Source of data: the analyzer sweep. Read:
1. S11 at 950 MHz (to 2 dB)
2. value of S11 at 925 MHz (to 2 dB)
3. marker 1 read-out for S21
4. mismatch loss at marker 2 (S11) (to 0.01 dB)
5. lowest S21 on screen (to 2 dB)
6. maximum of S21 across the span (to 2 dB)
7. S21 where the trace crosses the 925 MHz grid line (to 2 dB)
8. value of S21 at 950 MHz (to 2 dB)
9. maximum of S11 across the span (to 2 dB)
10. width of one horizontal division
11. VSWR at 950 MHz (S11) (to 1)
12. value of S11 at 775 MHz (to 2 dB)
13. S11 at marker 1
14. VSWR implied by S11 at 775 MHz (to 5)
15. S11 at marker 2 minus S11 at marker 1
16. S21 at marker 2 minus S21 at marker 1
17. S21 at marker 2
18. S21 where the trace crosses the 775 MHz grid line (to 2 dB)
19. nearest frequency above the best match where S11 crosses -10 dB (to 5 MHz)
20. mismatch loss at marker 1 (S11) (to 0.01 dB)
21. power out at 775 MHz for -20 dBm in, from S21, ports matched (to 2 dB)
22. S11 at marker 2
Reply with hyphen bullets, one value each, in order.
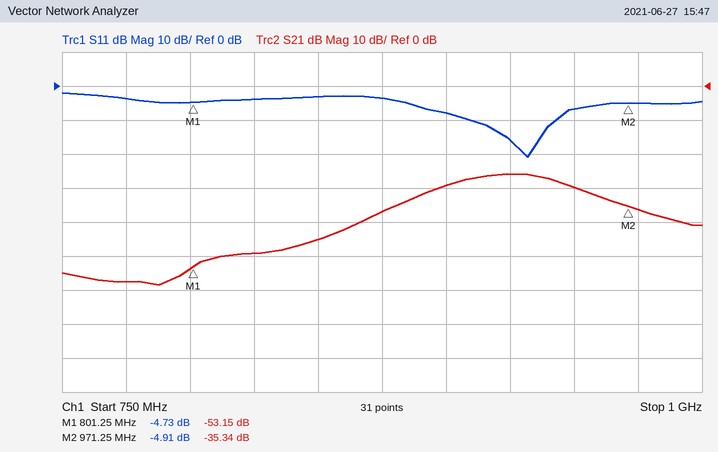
- -6 dB
- -16 dB
- -53.15 dB
- 1.69 dB
- -58 dB
- -26 dB
- -26 dB
- -30 dB
- -2 dB
- 25 MHz
- 3
- -4 dB
- -4.73 dB
- 5
- -0.18 dB
- 17.81 dB
- -35.34 dB
- -58 dB
- 945 MHz
- 1.78 dB
- -78 dBm
- -4.91 dB
